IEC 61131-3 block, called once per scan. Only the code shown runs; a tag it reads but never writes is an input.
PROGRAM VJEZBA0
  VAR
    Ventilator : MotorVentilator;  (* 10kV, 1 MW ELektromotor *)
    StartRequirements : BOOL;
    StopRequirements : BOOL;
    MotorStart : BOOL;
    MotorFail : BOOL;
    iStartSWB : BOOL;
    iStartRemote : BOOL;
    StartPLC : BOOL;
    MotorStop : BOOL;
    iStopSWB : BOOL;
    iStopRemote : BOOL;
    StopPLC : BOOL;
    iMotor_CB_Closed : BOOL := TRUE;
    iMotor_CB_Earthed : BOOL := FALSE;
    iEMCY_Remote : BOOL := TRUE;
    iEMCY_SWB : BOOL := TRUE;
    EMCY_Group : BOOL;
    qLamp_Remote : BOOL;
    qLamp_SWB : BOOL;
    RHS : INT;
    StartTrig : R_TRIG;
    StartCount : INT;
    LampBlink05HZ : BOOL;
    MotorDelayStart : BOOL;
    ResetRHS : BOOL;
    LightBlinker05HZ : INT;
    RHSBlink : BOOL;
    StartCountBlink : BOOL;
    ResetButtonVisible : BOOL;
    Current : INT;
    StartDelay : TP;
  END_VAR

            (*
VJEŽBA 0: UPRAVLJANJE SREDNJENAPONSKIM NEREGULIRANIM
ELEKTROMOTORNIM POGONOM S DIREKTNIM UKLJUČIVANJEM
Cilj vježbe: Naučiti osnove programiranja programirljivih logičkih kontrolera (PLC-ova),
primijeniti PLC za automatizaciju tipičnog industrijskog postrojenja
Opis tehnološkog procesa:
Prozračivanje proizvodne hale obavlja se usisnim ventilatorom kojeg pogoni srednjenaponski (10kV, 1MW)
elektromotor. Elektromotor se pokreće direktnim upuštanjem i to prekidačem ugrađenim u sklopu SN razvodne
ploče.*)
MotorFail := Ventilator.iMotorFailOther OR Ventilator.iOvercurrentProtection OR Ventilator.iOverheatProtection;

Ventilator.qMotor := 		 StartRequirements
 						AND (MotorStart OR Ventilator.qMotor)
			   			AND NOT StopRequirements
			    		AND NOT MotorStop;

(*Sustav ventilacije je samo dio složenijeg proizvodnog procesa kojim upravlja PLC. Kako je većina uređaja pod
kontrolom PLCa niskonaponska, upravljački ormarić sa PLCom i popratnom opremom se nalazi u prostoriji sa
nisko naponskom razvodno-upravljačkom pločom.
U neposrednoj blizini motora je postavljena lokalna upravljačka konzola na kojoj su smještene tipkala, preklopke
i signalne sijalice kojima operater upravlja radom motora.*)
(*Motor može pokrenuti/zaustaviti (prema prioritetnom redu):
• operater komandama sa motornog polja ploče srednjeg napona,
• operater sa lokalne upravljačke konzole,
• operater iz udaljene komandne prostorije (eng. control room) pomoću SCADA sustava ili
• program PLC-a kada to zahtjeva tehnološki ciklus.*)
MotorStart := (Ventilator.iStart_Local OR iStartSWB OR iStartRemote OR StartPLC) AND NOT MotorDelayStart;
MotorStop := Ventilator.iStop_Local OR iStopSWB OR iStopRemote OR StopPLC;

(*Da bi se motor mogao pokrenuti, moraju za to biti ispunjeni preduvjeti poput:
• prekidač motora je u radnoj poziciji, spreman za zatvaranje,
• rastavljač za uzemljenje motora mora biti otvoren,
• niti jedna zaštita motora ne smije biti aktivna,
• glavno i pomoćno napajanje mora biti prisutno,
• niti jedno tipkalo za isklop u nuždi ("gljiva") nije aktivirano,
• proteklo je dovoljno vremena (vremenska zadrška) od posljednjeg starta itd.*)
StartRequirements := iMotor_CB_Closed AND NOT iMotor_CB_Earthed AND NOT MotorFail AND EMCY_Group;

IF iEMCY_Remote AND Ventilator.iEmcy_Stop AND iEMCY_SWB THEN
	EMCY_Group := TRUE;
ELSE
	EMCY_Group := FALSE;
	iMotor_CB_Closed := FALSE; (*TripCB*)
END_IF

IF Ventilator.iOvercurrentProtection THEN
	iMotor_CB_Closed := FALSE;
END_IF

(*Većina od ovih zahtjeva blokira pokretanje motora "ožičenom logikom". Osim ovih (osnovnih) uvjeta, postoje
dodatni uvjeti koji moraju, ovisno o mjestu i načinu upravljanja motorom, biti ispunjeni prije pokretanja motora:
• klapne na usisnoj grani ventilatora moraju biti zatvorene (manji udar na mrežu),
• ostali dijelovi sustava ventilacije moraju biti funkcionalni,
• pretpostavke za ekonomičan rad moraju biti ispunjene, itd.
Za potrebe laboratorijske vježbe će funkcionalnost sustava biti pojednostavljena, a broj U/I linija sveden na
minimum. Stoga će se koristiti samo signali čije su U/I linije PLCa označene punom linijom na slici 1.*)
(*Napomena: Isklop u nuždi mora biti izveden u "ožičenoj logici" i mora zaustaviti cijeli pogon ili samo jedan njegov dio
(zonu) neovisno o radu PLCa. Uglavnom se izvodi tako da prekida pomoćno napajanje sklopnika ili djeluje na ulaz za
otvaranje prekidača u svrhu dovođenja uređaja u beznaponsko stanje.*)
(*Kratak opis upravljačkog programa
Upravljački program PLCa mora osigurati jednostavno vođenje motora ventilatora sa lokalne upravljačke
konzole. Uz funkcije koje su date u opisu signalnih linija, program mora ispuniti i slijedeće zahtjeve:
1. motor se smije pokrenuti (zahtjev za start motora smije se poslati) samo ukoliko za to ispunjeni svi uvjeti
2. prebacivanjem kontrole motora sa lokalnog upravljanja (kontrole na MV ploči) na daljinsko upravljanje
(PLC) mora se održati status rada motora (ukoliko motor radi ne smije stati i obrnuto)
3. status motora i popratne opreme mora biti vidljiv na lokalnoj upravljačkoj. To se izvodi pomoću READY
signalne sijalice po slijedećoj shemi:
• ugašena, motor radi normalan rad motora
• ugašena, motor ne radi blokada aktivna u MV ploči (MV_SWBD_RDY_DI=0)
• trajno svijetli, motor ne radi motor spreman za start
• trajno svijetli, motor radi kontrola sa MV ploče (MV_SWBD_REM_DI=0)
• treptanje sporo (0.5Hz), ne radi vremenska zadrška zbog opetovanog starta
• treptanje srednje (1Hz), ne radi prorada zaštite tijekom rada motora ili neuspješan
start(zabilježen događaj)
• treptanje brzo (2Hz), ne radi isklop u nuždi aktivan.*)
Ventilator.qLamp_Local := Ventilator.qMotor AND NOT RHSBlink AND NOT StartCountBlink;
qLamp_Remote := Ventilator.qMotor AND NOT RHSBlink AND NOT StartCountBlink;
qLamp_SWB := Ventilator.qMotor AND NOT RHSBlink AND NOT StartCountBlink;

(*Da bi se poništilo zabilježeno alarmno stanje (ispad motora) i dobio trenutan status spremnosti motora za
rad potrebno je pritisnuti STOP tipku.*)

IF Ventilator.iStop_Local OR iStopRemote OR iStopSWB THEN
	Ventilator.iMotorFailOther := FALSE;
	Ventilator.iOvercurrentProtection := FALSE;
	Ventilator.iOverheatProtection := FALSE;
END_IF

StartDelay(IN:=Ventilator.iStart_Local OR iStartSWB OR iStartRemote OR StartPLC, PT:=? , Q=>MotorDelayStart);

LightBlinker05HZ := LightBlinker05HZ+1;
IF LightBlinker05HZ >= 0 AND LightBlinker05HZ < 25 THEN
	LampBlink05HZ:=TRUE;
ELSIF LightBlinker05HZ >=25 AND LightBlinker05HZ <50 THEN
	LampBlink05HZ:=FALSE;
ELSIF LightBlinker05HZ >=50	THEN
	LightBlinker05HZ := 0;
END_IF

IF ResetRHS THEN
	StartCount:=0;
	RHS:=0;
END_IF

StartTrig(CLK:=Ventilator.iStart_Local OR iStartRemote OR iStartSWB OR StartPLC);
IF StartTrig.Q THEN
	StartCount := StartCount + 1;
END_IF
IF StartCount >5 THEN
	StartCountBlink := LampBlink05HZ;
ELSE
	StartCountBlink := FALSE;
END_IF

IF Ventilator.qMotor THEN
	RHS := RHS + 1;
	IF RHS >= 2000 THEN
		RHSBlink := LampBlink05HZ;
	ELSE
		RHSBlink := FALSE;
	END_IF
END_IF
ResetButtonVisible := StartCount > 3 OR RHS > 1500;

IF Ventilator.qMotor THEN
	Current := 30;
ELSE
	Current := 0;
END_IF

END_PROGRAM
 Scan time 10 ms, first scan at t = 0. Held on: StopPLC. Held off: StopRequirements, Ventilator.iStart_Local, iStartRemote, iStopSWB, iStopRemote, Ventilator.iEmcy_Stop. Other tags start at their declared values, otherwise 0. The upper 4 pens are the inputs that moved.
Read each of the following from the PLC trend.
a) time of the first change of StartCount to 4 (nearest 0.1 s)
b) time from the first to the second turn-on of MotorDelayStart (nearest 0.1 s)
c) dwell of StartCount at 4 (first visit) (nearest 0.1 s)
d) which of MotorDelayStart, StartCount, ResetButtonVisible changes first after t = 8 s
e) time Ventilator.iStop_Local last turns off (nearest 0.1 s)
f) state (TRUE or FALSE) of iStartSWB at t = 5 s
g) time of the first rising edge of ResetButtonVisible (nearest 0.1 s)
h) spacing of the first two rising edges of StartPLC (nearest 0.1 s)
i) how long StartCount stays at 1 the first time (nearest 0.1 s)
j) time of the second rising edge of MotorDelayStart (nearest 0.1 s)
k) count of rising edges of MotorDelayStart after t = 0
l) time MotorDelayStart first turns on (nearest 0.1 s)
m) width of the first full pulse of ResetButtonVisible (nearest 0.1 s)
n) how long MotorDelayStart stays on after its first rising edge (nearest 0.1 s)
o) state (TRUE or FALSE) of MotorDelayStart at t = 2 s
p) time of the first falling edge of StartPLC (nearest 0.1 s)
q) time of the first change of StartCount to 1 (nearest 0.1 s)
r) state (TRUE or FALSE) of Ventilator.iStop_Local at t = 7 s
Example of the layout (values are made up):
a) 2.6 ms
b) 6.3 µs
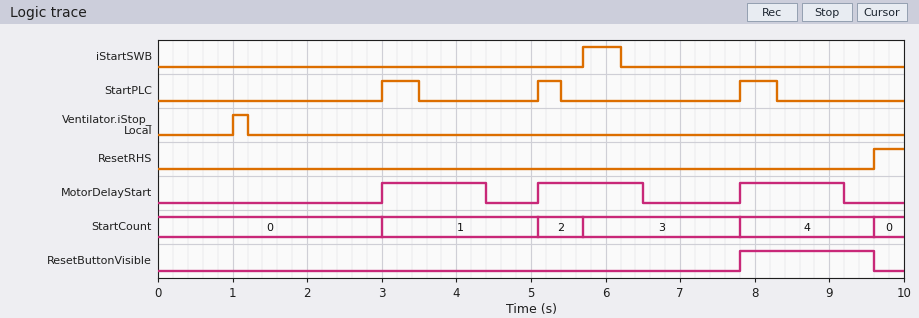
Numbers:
a) 7.8 s
b) 2.1 s
c) 1.8 s
d) MotorDelayStart
e) 1.2 s
f) FALSE
g) 7.8 s
h) 2.1 s
i) 2.1 s
j) 5.1 s
k) 3
l) 3.0 s
m) 1.8 s
n) 1.4 s
o) FALSE
p) 3.5 s
q) 3.0 s
r) FALSE
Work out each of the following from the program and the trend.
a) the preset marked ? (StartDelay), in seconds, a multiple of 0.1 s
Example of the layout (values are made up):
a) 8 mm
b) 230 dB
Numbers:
a) 1.4 s
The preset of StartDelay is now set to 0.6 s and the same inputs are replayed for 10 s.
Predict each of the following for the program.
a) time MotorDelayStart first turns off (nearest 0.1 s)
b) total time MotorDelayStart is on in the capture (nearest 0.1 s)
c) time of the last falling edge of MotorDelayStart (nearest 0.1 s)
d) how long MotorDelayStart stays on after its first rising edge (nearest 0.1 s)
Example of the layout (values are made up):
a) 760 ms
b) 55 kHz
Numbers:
a) 3.6 s
b) 1.8 s
c) 8.4 s
d) 0.6 s
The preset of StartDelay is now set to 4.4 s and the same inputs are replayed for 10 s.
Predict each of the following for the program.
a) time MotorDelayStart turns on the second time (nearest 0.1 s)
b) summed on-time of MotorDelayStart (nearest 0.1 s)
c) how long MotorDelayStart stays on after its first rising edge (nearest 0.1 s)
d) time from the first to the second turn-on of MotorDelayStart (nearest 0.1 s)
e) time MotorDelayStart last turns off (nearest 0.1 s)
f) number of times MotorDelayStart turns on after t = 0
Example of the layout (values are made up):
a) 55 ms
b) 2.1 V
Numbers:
a) 7.8 s
b) 6.6 s
c) 4.4 s
d) 4.8 s
e) 7.4 s
f) 2
